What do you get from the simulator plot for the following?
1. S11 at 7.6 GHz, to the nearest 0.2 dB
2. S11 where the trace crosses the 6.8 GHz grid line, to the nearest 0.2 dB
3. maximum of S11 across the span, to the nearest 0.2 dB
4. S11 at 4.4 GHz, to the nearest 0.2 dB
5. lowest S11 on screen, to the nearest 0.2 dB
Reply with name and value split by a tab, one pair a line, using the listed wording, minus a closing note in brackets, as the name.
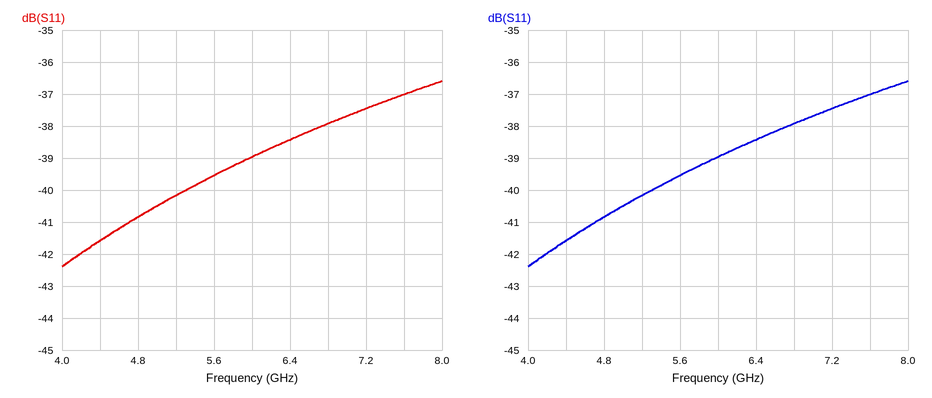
S11 at 7.6 GHz, to the nearest 0.2 dB	-37.0 dB
S11 where the trace crosses the 6.8 GHz grid line, to the nearest 0.2 dB	-38.0 dB
maximum of S11 across the span, to the nearest 0.2 dB	-36.6 dB
S11 at 4.4 GHz, to the nearest 0.2 dB	-41.6 dB
lowest S11 on screen, to the nearest 0.2 dB	-42.4 dB
